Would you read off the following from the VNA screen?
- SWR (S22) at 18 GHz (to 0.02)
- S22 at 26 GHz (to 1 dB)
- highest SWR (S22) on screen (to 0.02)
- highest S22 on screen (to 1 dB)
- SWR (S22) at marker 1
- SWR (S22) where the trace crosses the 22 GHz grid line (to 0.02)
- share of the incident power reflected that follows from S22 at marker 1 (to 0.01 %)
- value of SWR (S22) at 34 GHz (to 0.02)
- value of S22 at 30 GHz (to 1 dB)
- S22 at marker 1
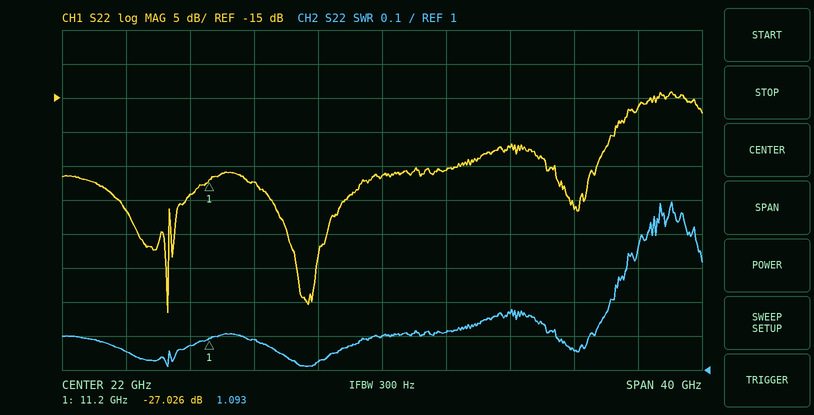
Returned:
1.02
-26 dB
1.50
-14 dB
1.093
1.10
0.20 %
1.06
-22 dB
-27.026 dB
